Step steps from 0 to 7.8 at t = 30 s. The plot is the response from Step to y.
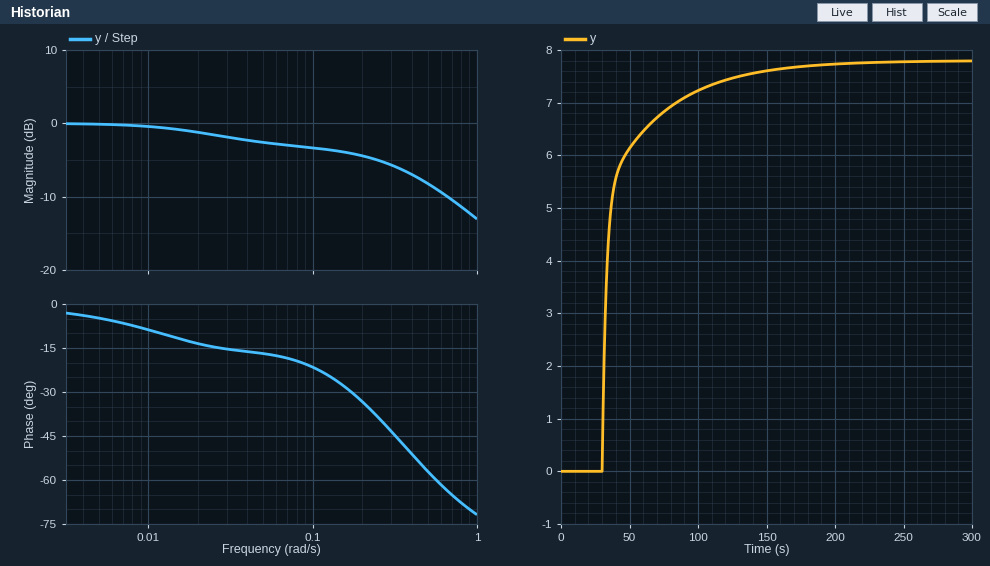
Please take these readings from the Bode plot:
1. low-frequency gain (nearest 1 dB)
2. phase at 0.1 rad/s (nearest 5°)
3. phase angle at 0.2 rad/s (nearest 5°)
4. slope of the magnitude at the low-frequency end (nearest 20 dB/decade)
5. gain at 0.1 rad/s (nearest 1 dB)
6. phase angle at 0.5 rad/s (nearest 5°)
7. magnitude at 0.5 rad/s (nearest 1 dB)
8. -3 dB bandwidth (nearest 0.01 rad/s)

0 dB
-20°
-35°
0 dB/decade
-3 dB
-55°
-8 dB
0.08 rad/s
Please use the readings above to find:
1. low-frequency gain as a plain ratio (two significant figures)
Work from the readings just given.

1.0
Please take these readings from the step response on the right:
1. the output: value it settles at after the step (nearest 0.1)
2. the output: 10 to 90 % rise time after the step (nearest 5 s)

7.8
55 s
